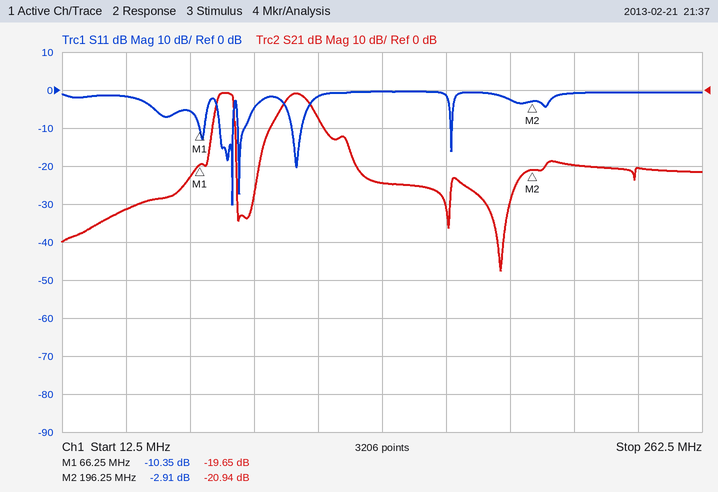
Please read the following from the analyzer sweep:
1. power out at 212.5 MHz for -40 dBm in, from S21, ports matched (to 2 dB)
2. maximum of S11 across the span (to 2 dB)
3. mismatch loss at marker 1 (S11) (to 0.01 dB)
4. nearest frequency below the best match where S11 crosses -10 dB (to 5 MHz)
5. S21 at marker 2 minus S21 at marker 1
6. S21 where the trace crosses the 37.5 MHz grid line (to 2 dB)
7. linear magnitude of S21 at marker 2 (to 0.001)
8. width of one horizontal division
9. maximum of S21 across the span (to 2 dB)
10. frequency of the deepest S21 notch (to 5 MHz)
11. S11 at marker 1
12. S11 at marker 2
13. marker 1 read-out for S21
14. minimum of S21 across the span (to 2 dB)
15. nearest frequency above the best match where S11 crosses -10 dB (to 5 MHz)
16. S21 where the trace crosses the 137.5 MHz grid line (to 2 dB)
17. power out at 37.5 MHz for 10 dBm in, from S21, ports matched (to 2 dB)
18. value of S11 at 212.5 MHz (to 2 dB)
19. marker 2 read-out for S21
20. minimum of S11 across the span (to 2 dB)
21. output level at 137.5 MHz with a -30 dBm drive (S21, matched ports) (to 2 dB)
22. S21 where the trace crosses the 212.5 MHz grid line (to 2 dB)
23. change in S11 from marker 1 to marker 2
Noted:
-60 dBm
0 dB
0.42 dB
75 MHz
-1.29 dB
-32 dB
0.090
25 MHz
0 dB
185 MHz
-10.35 dB
-2.91 dB
-19.65 dB
-48 dB
80 MHz
-24 dB
-22 dBm
0 dB
-20.94 dB
-30 dB
-54 dBm
-20 dB
7.44 dB
